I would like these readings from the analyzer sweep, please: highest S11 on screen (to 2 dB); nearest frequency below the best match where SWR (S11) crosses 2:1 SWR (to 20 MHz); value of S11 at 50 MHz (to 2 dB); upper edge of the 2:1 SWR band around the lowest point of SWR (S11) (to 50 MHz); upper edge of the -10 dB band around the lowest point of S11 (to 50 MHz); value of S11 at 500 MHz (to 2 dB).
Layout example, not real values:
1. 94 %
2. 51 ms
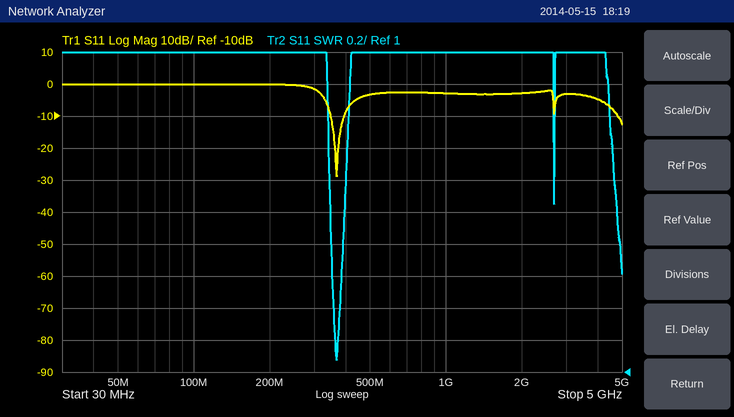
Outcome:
1. 0 dB
2. 340 MHz
3. 0 dB
4. 400 MHz
5. 400 MHz
6. -4 dB
